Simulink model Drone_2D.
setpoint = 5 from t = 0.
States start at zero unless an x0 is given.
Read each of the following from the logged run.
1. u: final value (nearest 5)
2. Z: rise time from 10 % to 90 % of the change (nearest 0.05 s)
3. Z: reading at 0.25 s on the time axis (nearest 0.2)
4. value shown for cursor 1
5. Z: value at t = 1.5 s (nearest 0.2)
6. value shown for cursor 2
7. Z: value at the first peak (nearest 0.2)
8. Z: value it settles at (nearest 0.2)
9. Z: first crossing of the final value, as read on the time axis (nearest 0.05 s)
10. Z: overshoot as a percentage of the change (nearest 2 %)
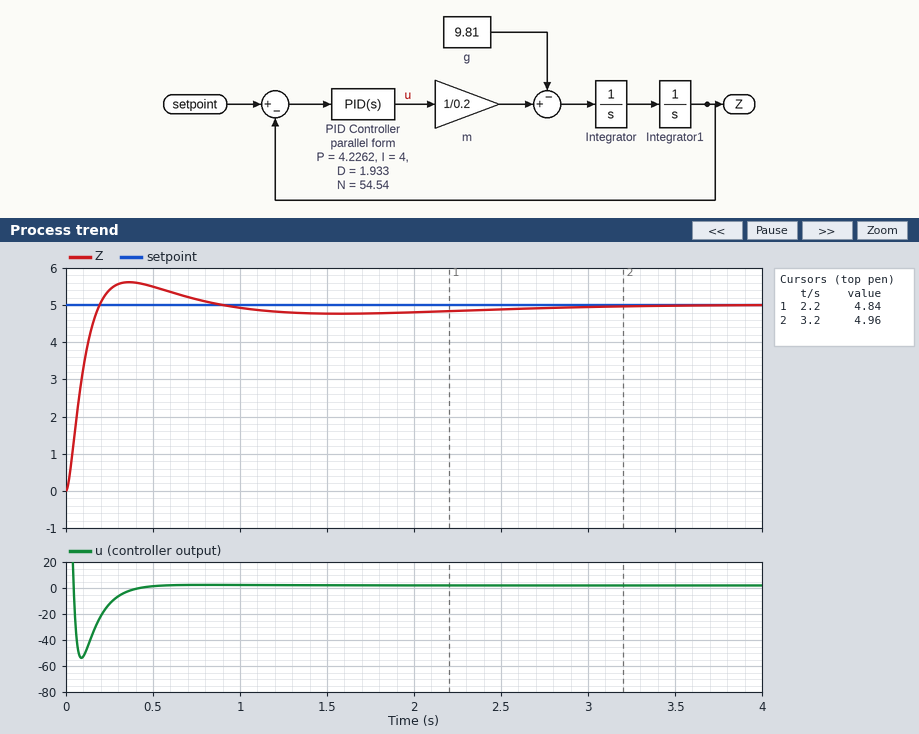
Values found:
0
0.15 s
5.4
4.84
4.8
4.96
5.6
5.0
0.20 s
12 %
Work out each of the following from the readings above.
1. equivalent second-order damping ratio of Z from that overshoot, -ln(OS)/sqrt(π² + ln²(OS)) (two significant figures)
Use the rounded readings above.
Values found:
0.56
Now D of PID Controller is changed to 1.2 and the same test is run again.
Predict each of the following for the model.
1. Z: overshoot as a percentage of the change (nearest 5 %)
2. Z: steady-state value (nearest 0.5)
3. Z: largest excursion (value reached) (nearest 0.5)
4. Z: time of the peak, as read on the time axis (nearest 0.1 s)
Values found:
25 %
5.0
6.0
0.5 s
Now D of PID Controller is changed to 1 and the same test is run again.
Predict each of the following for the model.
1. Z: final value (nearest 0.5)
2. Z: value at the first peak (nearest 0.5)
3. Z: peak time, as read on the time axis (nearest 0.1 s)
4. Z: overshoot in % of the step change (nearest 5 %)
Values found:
5.0
6.5
0.5 s
30 %
